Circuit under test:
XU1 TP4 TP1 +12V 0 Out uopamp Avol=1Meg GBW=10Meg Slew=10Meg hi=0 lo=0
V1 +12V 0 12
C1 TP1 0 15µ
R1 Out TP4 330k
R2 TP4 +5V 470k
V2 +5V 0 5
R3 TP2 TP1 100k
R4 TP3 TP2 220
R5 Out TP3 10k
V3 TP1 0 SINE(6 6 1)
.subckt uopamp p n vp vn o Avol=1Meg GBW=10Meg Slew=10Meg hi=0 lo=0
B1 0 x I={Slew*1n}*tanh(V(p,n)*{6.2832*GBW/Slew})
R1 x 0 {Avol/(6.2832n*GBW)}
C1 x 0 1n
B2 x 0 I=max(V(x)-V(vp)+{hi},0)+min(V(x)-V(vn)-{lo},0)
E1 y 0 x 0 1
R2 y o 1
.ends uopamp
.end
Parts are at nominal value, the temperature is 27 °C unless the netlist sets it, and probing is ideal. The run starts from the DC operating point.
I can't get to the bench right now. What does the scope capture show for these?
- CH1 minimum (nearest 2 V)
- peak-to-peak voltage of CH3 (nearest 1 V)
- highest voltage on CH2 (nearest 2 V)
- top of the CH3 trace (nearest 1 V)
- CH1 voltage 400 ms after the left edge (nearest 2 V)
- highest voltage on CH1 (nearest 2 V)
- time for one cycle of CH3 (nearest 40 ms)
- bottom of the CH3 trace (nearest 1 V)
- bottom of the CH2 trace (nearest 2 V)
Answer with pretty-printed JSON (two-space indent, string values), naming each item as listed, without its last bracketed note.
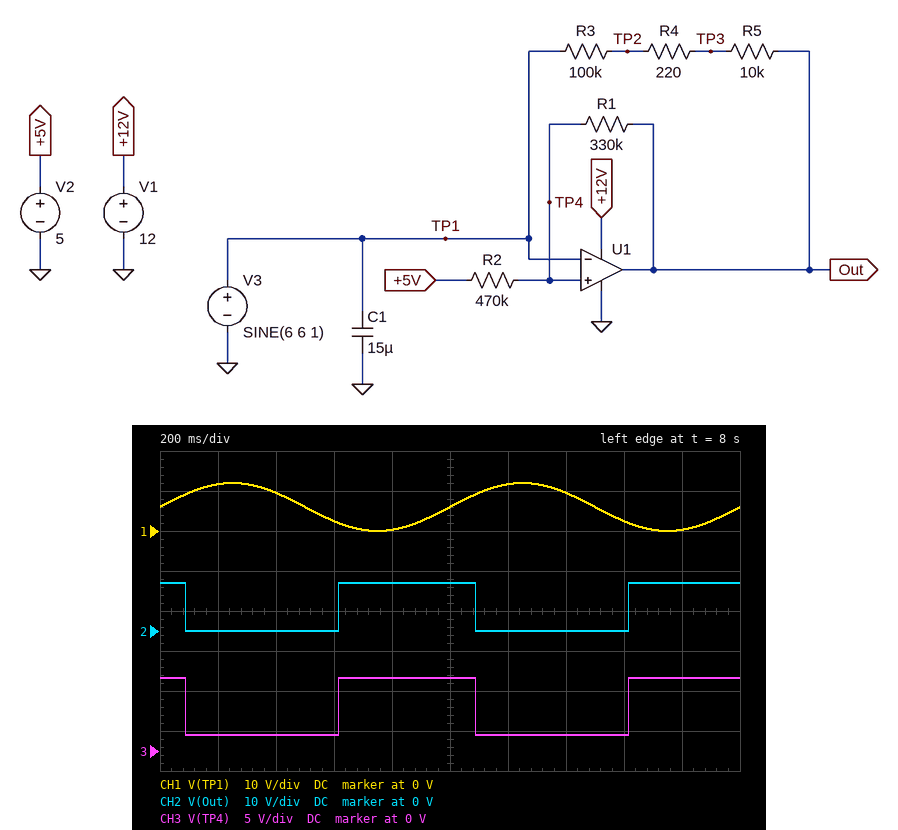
{
  "CH1 minimum": "0 V",
  "peak-to-peak voltage of CH3": "7 V",
  "highest voltage on CH2": "12 V",
  "top of the CH3 trace": "9 V",
  "CH1 voltage 400 ms after the left edge": "10 V",
  "highest voltage on CH1": "12 V",
  "time for one cycle of CH3": "1.00 s",
  "bottom of the CH3 trace": "2 V",
  "bottom of the CH2 trace": "0 V"
}
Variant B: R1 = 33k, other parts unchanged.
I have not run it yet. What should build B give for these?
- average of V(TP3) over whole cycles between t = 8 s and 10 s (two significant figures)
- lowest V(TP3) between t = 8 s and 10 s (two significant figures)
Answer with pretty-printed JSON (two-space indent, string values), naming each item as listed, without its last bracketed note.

{
  "average of V(TP3) over whole cycles between t = 8 s and 10 s": "5.9 V",
  "lowest V(TP3) between t = 8 s and 10 s": "30 mV"
}
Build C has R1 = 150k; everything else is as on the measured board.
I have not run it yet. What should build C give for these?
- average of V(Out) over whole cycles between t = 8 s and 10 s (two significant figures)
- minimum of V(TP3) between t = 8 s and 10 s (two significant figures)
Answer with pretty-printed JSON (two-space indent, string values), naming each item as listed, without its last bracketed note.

{
  "average of V(Out) over whole cycles between t = 8 s and 10 s": "5.8 V",
  "minimum of V(TP3) between t = 8 s and 10 s": "110 mV"
}
